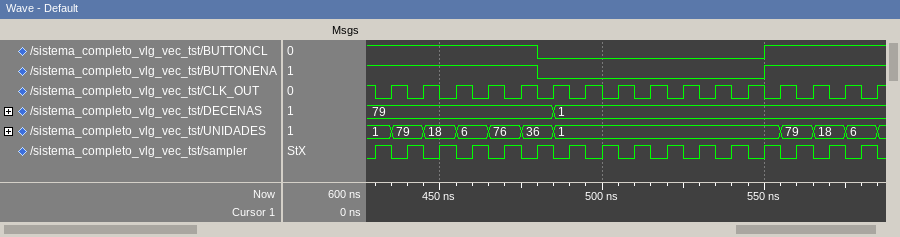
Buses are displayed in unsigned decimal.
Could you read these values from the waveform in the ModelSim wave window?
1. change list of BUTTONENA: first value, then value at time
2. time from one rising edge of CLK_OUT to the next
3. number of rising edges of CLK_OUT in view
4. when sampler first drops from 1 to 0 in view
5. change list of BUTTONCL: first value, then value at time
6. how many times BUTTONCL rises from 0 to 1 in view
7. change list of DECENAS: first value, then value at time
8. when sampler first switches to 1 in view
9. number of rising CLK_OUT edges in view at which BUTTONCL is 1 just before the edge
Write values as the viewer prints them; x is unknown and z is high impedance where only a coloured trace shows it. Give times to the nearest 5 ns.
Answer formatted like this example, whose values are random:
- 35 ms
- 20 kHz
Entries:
- 1, 0 at 480 ns, 1 at 550 ns
- 10 ns
- 16
- 435 ns
- 1, 0 at 480 ns, 1 at 550 ns
- 1
- 79, 1 at 485 ns
- 430 ns
- 9
